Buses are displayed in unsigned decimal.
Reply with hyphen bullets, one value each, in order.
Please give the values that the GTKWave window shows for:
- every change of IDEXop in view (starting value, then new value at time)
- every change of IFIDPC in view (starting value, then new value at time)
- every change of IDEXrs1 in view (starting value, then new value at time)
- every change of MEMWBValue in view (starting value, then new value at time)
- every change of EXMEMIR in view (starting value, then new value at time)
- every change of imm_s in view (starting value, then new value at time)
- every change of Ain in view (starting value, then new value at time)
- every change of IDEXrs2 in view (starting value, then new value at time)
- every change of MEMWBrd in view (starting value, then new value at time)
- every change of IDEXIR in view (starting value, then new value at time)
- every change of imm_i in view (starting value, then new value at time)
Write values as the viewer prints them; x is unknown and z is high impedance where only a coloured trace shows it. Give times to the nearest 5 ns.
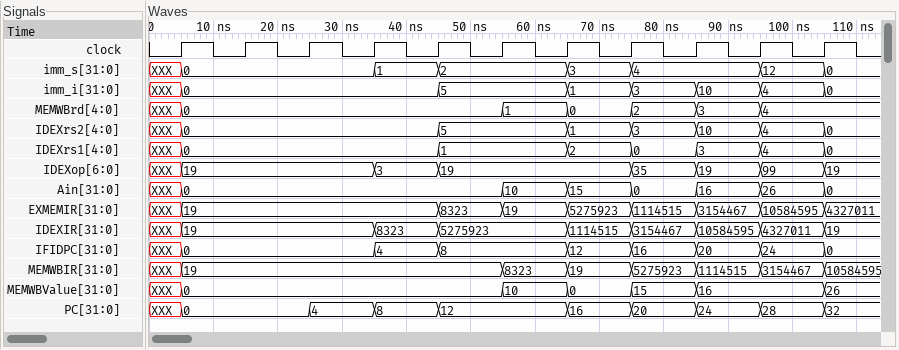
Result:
- XXX, 19 at 5 ns, 3 at 35 ns, 19 at 45 ns, 35 at 75 ns, 19 at 85 ns, 99 at 95 ns, 19 at 105 ns
- XXX, 0 at 5 ns, 4 at 35 ns, 8 at 45 ns, 12 at 65 ns, 16 at 75 ns, 20 at 85 ns, 24 at 95 ns, 0 at 105 ns
- XXX, 0 at 5 ns, 1 at 45 ns, 2 at 65 ns, 0 at 75 ns, 3 at 85 ns, 4 at 95 ns, 0 at 105 ns
- XXX, 0 at 5 ns, 10 at 55 ns, 0 at 65 ns, 15 at 75 ns, 16 at 85 ns, 26 at 105 ns
- XXX, 19 at 5 ns, 8323 at 45 ns, 19 at 55 ns, 5275923 at 65 ns, 1114515 at 75 ns, 3154467 at 85 ns, 10584595 at 95 ns, 4327011 at 105 ns
- XXX, 0 at 5 ns, 1 at 35 ns, 2 at 45 ns, 3 at 65 ns, 4 at 75 ns, 12 at 95 ns, 0 at 105 ns
- XXX, 0 at 5 ns, 10 at 55 ns, 15 at 65 ns, 0 at 75 ns, 16 at 85 ns, 26 at 95 ns, 0 at 105 ns
- XXX, 0 at 5 ns, 5 at 45 ns, 1 at 65 ns, 3 at 75 ns, 10 at 85 ns, 4 at 95 ns, 0 at 105 ns
- XXX, 0 at 5 ns, 1 at 55 ns, 0 at 65 ns, 2 at 75 ns, 3 at 85 ns, 4 at 95 ns
- XXX, 19 at 5 ns, 8323 at 35 ns, 5275923 at 45 ns, 1114515 at 65 ns, 3154467 at 75 ns, 10584595 at 85 ns, 4327011 at 95 ns, 19 at 105 ns
- XXX, 0 at 5 ns, 5 at 45 ns, 1 at 65 ns, 3 at 75 ns, 10 at 85 ns, 4 at 95 ns, 0 at 105 ns
